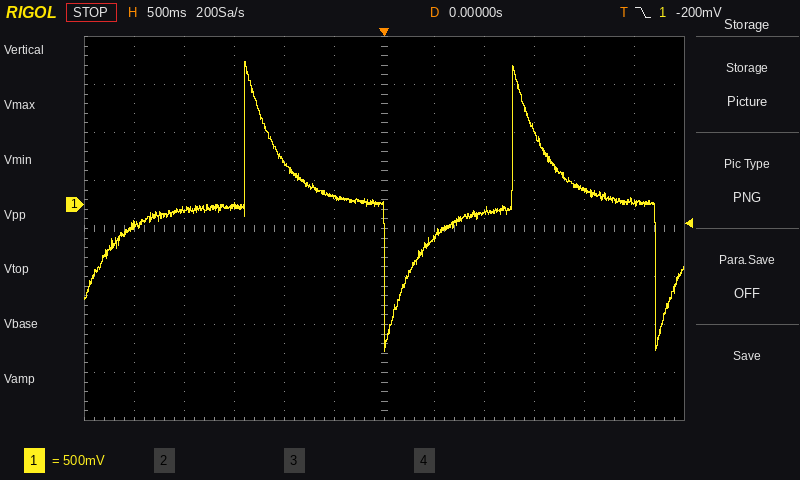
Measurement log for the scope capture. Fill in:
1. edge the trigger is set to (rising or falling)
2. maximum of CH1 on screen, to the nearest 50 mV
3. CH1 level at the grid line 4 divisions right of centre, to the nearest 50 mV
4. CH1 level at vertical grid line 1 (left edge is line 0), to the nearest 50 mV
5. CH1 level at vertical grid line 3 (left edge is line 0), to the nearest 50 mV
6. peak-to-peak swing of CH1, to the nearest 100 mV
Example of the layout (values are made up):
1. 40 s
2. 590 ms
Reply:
1. falling
2. 1.50 V
3. 150 mV
4. -200 mV
5. 0 mV
6. 3.00 V
